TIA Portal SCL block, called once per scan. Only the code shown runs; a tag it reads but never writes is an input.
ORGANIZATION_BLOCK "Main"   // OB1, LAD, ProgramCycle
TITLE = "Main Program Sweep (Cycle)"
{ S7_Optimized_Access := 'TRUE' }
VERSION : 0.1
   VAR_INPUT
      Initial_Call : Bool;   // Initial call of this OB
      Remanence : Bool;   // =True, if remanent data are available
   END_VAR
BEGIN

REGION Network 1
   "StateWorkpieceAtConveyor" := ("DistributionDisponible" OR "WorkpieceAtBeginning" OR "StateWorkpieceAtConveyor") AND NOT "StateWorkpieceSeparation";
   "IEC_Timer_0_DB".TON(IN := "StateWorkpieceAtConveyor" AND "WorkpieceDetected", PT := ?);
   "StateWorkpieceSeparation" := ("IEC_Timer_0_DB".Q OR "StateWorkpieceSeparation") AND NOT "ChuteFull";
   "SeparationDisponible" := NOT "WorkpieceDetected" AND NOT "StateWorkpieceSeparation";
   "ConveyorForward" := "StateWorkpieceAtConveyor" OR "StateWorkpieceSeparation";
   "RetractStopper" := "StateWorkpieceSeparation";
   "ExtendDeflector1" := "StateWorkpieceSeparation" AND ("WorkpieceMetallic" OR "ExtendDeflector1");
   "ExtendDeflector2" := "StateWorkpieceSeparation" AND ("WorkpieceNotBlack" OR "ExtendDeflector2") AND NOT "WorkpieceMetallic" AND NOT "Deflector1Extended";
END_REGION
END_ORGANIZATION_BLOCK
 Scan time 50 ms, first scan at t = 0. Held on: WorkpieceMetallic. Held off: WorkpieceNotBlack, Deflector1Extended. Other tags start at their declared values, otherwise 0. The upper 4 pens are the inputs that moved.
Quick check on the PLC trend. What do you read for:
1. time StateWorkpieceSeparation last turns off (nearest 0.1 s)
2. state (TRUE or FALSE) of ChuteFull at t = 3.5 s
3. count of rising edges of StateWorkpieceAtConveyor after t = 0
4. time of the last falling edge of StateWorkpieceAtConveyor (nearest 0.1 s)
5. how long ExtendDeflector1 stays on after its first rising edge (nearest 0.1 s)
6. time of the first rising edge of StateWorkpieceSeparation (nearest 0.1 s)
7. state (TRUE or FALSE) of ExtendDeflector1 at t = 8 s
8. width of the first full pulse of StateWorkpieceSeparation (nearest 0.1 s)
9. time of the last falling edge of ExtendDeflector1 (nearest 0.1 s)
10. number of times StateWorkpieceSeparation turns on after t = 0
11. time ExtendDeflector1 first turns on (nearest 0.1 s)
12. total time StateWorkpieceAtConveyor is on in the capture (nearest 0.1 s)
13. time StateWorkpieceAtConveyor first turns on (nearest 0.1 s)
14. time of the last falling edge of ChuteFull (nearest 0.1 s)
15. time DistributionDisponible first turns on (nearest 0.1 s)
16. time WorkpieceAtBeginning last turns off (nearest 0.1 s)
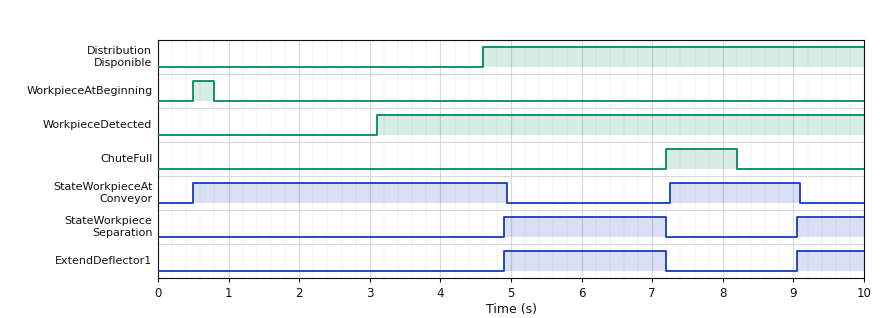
7.2 s
FALSE
2
9.1 s
2.3 s
4.9 s
FALSE
2.3 s
7.2 s
2
4.9 s
6.3 s
0.5 s
8.2 s
4.6 s
0.8 s
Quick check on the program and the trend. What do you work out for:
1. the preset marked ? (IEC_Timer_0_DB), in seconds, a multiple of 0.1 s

1.8 s
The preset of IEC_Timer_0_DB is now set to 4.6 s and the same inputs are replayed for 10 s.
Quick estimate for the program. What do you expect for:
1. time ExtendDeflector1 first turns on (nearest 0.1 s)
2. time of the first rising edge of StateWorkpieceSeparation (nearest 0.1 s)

8.2 s
8.2 s
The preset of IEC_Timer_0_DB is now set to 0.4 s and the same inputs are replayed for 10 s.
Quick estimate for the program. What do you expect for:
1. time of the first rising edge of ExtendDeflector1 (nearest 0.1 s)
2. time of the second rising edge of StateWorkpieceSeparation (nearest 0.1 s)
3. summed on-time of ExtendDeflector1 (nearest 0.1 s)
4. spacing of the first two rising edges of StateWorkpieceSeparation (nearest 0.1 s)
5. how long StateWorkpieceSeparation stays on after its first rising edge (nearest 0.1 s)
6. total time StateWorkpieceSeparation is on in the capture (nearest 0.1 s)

3.5 s
8.2 s
5.5 s
4.7 s
3.7 s
5.5 s
